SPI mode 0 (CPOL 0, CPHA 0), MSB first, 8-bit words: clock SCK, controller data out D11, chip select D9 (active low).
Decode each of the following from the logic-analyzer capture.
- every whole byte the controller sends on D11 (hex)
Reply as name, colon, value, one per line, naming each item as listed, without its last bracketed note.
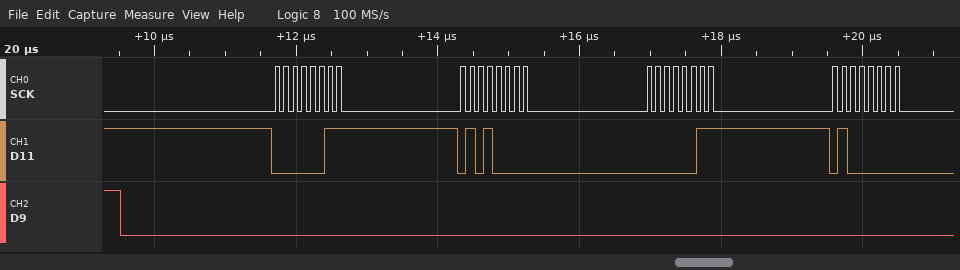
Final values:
every whole byte the controller sends on D11: 03 50 03 40
